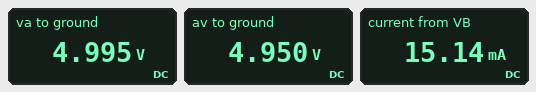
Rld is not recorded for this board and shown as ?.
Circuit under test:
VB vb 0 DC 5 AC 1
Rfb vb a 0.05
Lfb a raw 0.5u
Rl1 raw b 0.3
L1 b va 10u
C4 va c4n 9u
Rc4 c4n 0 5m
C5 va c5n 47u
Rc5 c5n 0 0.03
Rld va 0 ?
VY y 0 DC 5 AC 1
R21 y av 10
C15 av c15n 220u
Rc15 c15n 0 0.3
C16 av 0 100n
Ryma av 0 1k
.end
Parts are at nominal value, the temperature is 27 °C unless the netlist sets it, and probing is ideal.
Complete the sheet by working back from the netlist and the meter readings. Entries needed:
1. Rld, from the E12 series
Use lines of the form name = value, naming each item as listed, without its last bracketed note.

Rld, from the E12 series = 330 Ω
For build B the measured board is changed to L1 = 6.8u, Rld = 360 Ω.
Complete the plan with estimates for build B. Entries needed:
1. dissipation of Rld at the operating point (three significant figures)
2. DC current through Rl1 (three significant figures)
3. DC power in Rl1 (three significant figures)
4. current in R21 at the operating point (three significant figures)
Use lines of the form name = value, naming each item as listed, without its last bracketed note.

dissipation of Rld at the operating point = 69.3 mW
DC current through Rl1 = 13.9 mA
DC power in Rl1 = 57.8 µW
current in R21 at the operating point = 4.95 mA
